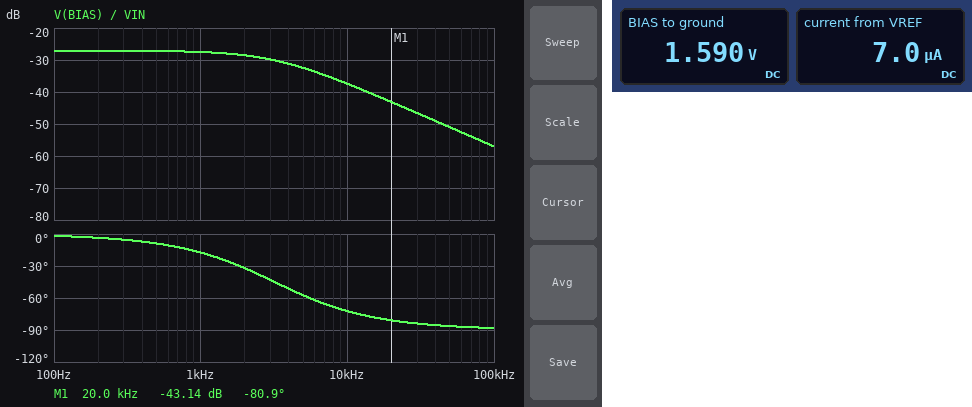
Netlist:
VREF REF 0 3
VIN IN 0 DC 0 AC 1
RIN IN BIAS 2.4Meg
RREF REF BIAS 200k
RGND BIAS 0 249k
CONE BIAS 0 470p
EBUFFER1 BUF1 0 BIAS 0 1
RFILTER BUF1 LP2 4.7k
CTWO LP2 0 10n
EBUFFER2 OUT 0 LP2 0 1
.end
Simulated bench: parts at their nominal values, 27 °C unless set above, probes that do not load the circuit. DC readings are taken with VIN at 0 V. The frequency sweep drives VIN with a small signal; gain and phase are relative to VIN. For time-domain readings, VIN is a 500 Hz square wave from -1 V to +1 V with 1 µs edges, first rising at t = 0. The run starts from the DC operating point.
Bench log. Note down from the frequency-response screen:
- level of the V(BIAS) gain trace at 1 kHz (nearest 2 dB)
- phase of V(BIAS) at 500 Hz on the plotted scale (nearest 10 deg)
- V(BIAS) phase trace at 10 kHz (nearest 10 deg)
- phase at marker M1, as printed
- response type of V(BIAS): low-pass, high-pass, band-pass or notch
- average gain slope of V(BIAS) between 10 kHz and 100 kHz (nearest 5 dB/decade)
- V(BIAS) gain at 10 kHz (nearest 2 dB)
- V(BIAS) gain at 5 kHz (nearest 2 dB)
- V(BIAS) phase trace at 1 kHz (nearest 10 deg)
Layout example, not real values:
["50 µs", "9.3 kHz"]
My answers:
["-28 dB", "-10 deg", "-70 deg", "-80.9 deg", "low-pass", "-20 dB/decade", "-38 dB", "-32 dB", "-20 deg"]
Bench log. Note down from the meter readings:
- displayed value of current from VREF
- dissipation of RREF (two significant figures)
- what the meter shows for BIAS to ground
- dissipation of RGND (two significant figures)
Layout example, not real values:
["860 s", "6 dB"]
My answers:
["7.0 µA", "9.9 µW", "1.590 V", "10 µW"]
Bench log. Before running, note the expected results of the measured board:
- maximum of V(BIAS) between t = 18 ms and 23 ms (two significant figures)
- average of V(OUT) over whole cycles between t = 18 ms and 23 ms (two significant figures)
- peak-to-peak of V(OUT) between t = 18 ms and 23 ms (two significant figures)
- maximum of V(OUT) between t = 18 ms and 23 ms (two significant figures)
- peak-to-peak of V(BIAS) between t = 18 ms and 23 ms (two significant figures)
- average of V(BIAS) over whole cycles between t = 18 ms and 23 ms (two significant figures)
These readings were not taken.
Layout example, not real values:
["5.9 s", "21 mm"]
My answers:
["1.6 V", "1.6 V", "88 mV", "1.6 V", "88 mV", "1.6 V"]
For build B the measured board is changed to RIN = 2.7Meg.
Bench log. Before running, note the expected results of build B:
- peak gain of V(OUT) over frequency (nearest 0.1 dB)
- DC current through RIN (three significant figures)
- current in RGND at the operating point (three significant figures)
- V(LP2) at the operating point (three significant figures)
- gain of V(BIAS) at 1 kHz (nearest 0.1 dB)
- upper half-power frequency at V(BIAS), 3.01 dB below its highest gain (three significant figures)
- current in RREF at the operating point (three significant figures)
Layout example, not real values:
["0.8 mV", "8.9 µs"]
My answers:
["-28.1 dB", "592 nA", "6.42 µA", "1.60 V", "-28.5 dB", "3.18 kHz", "7.01 µA"]
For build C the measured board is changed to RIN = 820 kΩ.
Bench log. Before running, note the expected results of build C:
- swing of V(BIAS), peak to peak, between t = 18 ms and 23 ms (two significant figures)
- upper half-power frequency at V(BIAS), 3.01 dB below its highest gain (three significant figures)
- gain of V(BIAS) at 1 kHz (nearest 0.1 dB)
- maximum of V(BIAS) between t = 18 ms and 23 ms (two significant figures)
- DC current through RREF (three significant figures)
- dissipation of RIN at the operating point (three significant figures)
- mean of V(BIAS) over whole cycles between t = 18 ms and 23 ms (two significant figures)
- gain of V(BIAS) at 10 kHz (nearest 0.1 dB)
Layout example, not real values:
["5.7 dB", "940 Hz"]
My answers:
["240 mV", "3.47 kHz", "-18.8 dB", "1.6 V", "7.67 µA", "2.62 µW", "1.5 V", "-28.2 dB"]
